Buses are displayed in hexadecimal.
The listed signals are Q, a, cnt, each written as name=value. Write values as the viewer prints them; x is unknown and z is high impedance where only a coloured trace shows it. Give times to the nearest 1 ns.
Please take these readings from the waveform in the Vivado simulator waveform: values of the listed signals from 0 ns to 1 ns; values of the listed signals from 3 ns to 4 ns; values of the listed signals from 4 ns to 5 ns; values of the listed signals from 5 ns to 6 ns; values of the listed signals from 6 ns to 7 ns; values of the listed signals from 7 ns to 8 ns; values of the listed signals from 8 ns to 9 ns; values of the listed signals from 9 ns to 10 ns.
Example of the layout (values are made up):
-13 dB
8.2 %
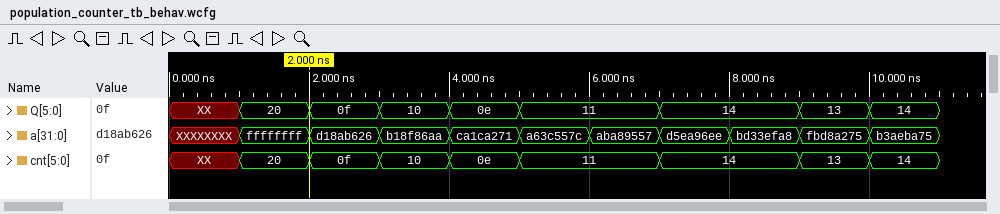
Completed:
Q=XX, a=XXXXXXXX, cnt=XX
Q=10, a=b18f86aa, cnt=10
Q=0e, a=ca1ca271, cnt=0e
Q=11, a=a63c557c, cnt=11
Q=11, a=aba89557, cnt=11
Q=14, a=d5ea96ee, cnt=14
Q=14, a=bd33efa8, cnt=14
Q=13, a=fbd8a275, cnt=13
